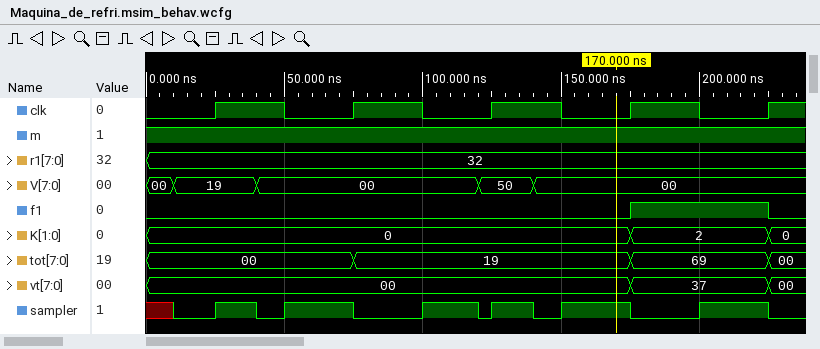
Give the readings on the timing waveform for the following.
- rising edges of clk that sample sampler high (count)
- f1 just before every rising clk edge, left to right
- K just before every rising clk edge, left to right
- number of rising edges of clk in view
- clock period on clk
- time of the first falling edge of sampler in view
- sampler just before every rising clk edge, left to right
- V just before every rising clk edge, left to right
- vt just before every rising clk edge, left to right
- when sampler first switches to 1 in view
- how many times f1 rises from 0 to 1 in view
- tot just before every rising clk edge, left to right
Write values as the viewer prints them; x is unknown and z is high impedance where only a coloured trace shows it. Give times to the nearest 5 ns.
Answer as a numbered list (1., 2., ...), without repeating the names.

1. 3
2. 0 0 0 0 1
3. 0, 0, 0, 0, 2
4. 5
5. 50 ns
6. 40 ns
7. 0 1 0 1 1
8. 19, 00, 50, 00, 00
9. 00, 00, 00, 00, 37
10. 25 ns
11. 1
12. 00, 00, 19, 19, 69
